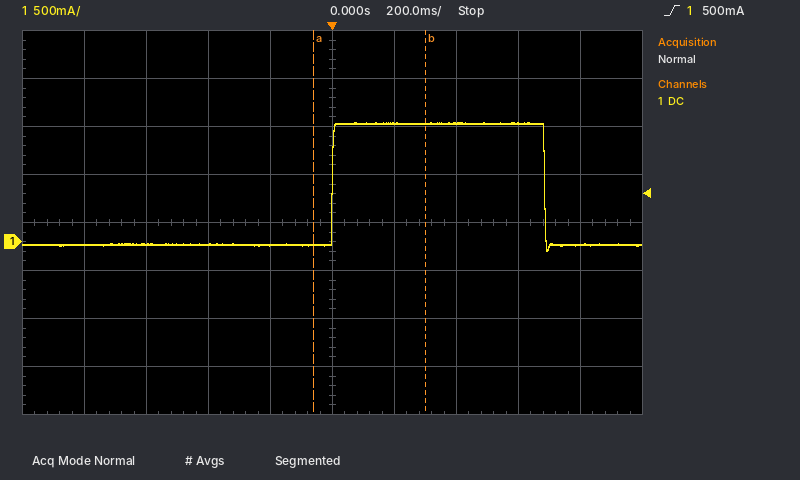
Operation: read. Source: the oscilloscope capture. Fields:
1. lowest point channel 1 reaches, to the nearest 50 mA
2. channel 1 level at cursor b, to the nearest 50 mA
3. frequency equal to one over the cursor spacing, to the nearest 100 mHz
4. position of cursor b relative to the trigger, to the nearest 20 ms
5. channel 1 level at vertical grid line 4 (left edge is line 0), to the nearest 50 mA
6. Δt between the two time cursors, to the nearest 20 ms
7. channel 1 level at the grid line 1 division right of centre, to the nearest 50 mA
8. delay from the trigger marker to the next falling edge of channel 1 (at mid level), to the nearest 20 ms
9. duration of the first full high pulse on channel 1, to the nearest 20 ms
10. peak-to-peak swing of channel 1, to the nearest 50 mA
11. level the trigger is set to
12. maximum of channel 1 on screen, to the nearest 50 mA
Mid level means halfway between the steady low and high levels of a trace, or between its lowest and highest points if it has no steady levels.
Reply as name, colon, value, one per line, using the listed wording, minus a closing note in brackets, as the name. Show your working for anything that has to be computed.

lowest point channel 1 reaches, to the nearest 50 mA: -100 mA
channel 1 level at cursor b, to the nearest 50 mA: 1.25 A
frequency equal to one over the cursor spacing, to the nearest 100 mHz: 1 / 360 ms ≈ 2.8 Hz
position of cursor b relative to the trigger, to the nearest 20 ms: +300 ms
channel 1 level at vertical grid line 4 (left edge is line 0), to the nearest 50 mA: -50 mA
Δt between the two time cursors, to the nearest 20 ms: 360 ms
channel 1 level at the grid line 1 division right of centre, to the nearest 50 mA: 1.25 A
delay from the trigger marker to the next falling edge of channel 1 (at mid level), to the nearest 20 ms: 680 ms
duration of the first full high pulse on channel 1, to the nearest 20 ms: 680 ms
peak-to-peak swing of channel 1, to the nearest 50 mA: 1.25 A − (-100 mA) = 1.35 A
level the trigger is set to: 500 mA
maximum of channel 1 on screen, to the nearest 50 mA: 1.25 A
